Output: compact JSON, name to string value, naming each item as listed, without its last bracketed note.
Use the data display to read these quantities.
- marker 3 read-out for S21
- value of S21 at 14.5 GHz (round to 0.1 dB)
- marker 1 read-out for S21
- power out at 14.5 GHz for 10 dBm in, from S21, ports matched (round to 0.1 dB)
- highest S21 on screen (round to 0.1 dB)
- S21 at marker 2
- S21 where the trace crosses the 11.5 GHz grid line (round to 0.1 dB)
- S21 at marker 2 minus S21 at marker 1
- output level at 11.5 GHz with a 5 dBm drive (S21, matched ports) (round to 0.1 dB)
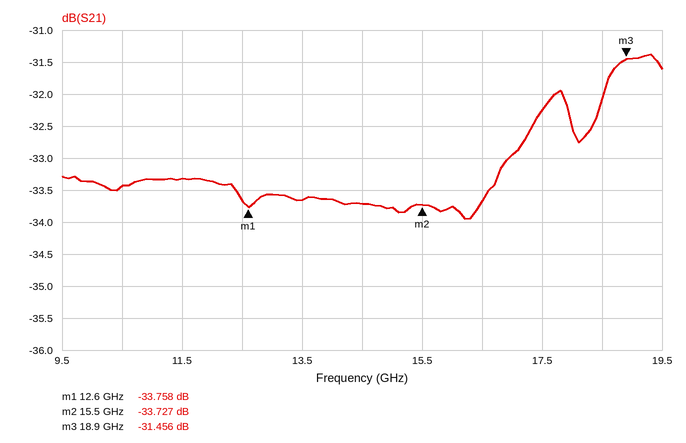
{"marker 3 read-out for S21": "-31.456 dB", "value of S21 at 14.5 GHz": "-33.7 dB", "marker 1 read-out for S21": "-33.758 dB", "power out at 14.5 GHz for 10 dBm in, from S21, ports matched": "-23.7 dBm", "highest S21 on screen": "-31.4 dB", "S21 at marker 2": "-33.727 dB", "S21 where the trace crosses the 11.5 GHz grid line": "-33.3 dB", "S21 at marker 2 minus S21 at marker 1": "0.031 dB", "output level at 11.5 GHz with a 5 dBm drive (S21, matched ports)": "-28.3 dBm"}
